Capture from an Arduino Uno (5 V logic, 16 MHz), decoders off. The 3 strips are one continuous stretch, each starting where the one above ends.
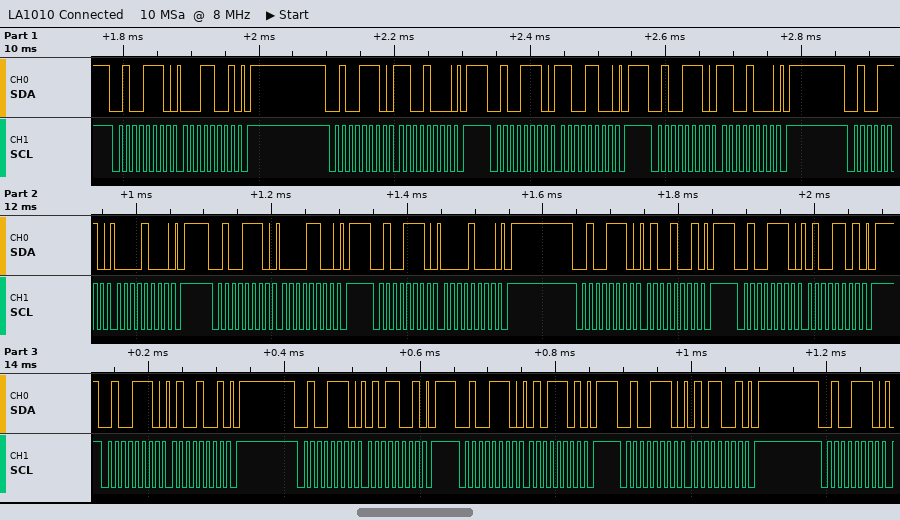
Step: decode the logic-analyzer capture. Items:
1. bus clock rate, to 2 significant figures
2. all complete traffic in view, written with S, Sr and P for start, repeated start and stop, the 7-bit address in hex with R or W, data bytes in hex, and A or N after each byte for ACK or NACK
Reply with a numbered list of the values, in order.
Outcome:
1. 100 kHz
2. S 27W A 19 A P S 27W A C8 A P S 27W A CC A P S 27W A C8 A P S 27W A 08 A P S 27W A 0C A P S 27W A 08 A P S 27W A 49 A P S 27W A 4D A P S 27W A 49 A P S 27W A 59 A P S 27W A 5D A P S 27W A 59 A P S 27W A
